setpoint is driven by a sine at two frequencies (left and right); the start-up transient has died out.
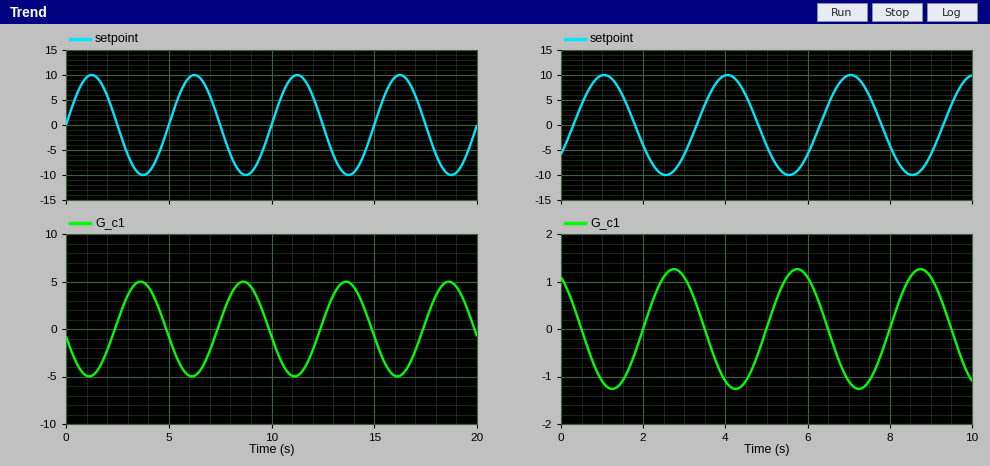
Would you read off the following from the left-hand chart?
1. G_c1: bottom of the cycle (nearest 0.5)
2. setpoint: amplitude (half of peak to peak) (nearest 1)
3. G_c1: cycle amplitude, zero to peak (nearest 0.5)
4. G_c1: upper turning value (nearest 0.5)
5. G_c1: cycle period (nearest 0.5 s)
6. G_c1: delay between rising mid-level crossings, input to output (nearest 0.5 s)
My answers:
-5.0
10
5.0
5.0
5.0 s
2.5 s
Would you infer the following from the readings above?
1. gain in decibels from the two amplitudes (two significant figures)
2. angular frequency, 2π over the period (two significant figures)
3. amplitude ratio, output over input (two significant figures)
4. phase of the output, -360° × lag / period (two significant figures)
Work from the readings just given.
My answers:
-6.0 dB
1.3 rad/s
0.50
-180°
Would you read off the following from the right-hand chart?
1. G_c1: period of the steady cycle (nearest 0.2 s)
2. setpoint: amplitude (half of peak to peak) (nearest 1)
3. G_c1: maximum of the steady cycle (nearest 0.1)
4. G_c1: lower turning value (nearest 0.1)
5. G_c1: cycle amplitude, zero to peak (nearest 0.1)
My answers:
3.0 s
10
1.3
-1.3
1.3
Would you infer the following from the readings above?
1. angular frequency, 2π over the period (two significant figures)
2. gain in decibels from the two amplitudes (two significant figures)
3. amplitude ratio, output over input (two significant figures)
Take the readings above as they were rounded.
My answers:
2.1 rad/s
-18 dB
0.13
